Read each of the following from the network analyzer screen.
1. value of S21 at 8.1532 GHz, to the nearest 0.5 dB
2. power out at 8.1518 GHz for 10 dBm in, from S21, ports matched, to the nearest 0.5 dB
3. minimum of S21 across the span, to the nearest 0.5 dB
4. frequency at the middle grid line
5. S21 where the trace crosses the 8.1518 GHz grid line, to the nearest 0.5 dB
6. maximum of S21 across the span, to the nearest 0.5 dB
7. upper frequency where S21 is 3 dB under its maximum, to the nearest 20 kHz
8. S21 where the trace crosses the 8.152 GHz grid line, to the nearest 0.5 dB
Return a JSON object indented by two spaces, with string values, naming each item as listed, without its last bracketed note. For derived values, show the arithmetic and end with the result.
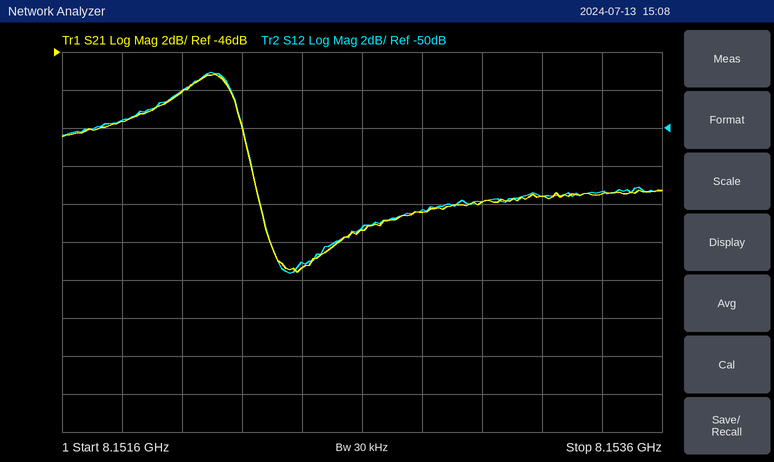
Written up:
{
  "value of S21 at 8.1532 GHz, to the nearest 0.5 dB": "-53.5 dB",
  "power out at 8.1518 GHz for 10 dBm in, from S21, ports matched, to the nearest 0.5 dB": "10 dBm + (-49.5 dB) = -39.5 dBm",
  "minimum of S21 across the span, to the nearest 0.5 dB": "-57.5 dB",
  "frequency at the middle grid line": "8.1526 GHz",
  "S21 where the trace crosses the 8.1518 GHz grid line, to the nearest 0.5 dB": "-49.5 dB",
  "maximum of S21 across the span, to the nearest 0.5 dB": "-47.0 dB",
  "upper frequency where S21 is 3 dB under its maximum, to the nearest 20 kHz": "8.15220 GHz",
  "S21 where the trace crosses the 8.152 GHz grid line, to the nearest 0.5 dB": "-48.0 dB"
}
